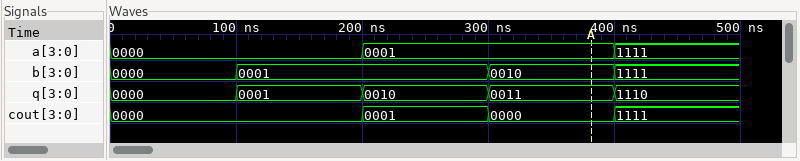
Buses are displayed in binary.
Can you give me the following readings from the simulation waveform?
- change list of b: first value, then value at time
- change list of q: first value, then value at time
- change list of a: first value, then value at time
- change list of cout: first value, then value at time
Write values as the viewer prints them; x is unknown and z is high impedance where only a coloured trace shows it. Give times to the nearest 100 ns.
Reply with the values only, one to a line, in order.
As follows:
0000, 0001 at 100 ns, 0010 at 300 ns, 1111 at 400 ns
0000, 0001 at 100 ns, 0010 at 200 ns, 0011 at 300 ns, 1110 at 400 ns
0000, 0001 at 200 ns, 1111 at 400 ns
0000, 0001 at 200 ns, 0000 at 300 ns, 1111 at 400 ns
